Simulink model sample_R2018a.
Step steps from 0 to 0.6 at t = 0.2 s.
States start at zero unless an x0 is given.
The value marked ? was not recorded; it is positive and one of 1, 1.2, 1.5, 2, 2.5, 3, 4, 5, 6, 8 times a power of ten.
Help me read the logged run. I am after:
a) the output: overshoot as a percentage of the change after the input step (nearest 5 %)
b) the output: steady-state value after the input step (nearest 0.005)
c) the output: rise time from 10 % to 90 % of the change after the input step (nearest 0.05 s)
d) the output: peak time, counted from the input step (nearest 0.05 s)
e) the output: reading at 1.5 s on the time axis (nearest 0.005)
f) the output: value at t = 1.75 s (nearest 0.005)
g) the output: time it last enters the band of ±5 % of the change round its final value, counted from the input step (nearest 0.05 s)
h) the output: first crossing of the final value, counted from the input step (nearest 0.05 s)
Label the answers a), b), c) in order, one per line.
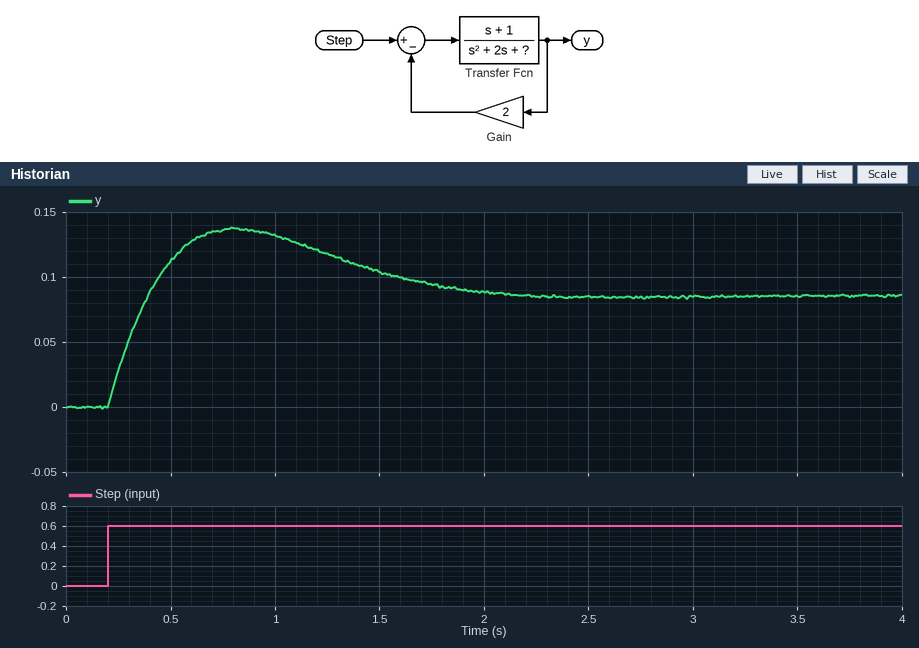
a) 60 %
b) 0.085
c) 0.15 s
d) 0.60 s
e) 0.105
f) 0.095
g) 1.70 s
h) 0.20 s
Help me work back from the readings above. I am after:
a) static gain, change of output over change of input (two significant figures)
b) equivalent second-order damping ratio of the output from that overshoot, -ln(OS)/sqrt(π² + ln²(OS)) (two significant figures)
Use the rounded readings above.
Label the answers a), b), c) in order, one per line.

a) 0.14
b) 0.16
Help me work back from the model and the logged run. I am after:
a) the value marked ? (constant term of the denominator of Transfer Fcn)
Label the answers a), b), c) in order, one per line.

a) 5
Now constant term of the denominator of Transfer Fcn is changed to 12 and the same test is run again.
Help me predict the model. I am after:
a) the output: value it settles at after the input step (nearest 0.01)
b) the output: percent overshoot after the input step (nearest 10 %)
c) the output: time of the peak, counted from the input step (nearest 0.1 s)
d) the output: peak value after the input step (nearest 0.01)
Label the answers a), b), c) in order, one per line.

a) 0.04
b) 150 %
c) 0.4 s
d) 0.11
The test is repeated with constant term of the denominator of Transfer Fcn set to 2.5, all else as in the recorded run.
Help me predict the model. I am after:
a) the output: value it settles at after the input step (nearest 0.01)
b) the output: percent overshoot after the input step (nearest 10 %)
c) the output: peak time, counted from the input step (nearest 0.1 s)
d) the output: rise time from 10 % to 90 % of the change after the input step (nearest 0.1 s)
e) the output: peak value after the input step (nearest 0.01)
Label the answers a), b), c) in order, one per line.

a) 0.13
b) 20 %
c) 0.9 s
d) 0.3 s
e) 0.16
